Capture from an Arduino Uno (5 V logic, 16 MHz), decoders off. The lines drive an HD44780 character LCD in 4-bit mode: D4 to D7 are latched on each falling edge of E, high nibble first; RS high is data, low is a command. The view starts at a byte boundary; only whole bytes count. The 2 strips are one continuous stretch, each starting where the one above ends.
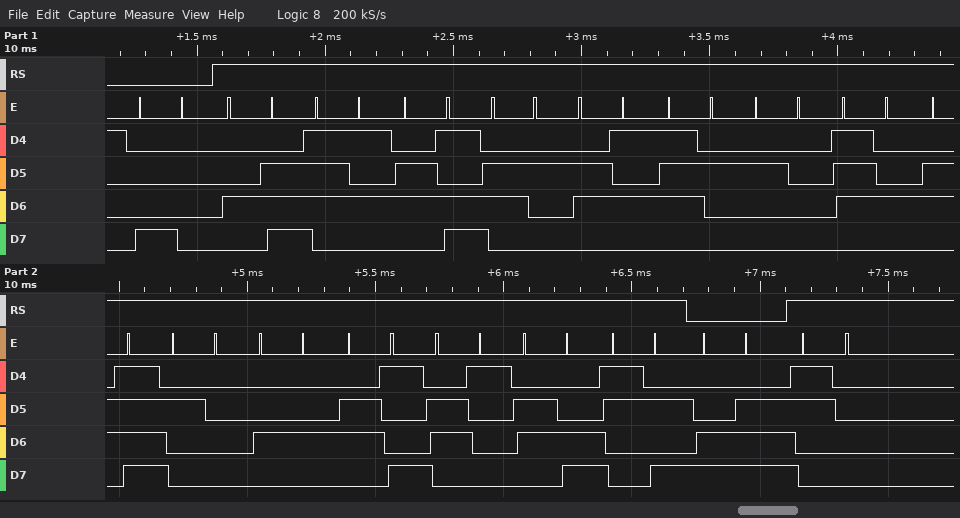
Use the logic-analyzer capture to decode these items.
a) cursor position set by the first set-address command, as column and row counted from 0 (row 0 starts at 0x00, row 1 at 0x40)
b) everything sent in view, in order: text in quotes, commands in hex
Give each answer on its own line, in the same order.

column 0, row 0
0x80 "Number to Dial:" 0xCE "0"
